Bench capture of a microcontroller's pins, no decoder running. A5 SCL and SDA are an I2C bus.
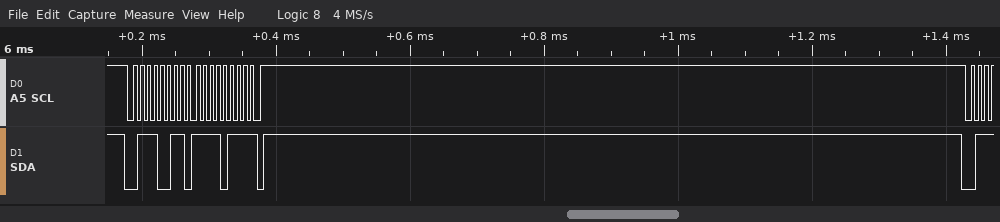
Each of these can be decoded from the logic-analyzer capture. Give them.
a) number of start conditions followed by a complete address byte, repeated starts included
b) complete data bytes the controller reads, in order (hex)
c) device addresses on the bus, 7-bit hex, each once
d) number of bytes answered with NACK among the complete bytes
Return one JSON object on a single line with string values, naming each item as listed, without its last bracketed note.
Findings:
{"number of start conditions followed by a complete address byte, repeated starts included": "1", "complete data bytes the controller reads, in order": "F7", "device addresses on the bus, 7-bit hex, each once": "0x39", "number of bytes answered with NACK among the complete bytes": "1"}
